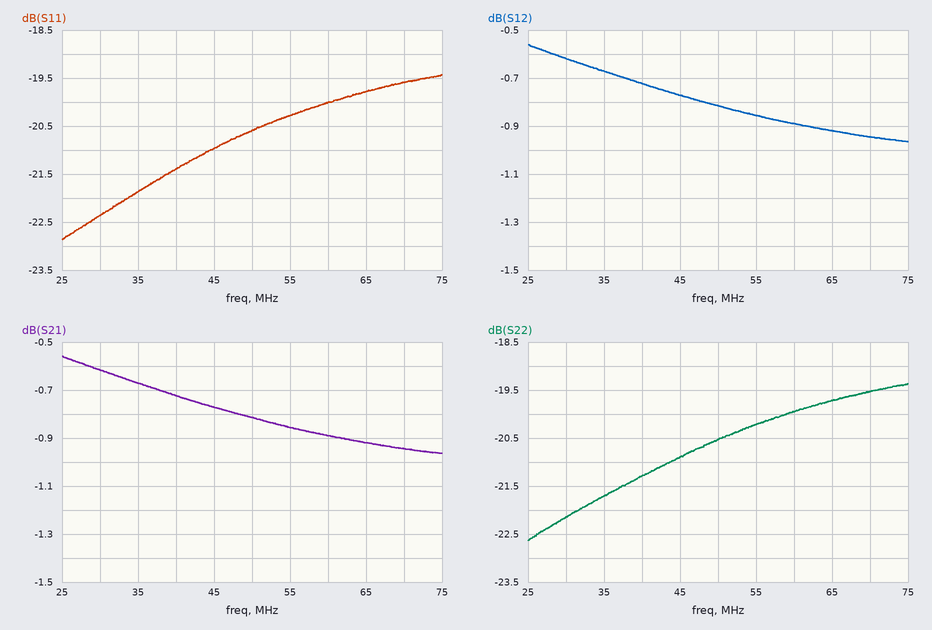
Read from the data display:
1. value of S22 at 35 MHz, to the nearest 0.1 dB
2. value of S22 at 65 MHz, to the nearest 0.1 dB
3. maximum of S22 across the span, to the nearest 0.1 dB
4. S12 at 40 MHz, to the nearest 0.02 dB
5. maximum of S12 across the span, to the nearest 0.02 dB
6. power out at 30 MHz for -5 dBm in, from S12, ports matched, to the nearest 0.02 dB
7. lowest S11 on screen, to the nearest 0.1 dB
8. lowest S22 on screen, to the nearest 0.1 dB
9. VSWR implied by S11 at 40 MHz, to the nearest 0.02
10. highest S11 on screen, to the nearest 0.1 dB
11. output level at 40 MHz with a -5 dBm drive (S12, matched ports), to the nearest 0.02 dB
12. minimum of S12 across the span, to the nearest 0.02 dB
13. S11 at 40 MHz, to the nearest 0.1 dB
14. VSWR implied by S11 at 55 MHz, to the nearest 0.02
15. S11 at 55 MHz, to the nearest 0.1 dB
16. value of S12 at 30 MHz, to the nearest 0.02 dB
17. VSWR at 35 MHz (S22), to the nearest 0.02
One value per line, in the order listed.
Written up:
-21.7 dB
-19.7 dB
-19.4 dB
-0.72 dB
-0.56 dB
-5.62 dBm
-22.9 dB
-22.6 dB
1.18
-19.4 dB
-5.72 dBm
-0.96 dB
-21.4 dB
1.22
-20.3 dB
-0.62 dB
1.18
